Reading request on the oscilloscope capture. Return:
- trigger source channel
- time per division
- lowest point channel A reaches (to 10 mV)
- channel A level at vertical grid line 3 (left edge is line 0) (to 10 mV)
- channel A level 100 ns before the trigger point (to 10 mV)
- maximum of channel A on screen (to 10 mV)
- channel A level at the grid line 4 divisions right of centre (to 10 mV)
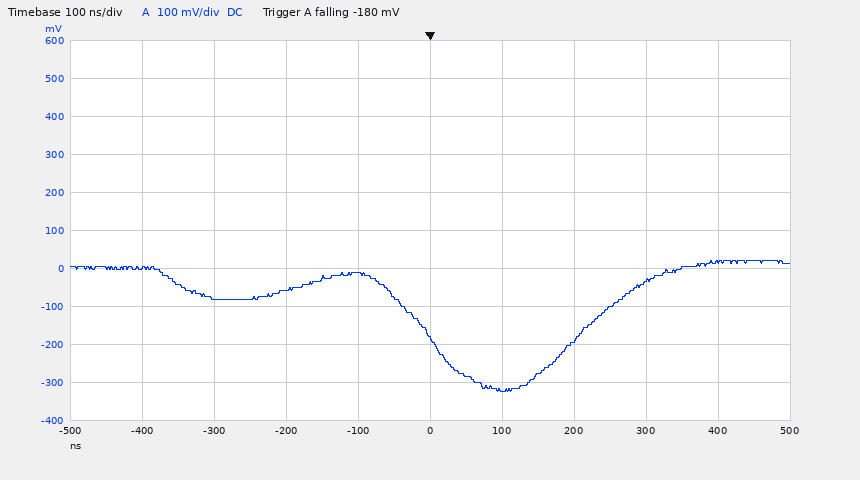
channel A
100 ns
-320 mV
-60 mV
-10 mV
20 mV
20 mV
